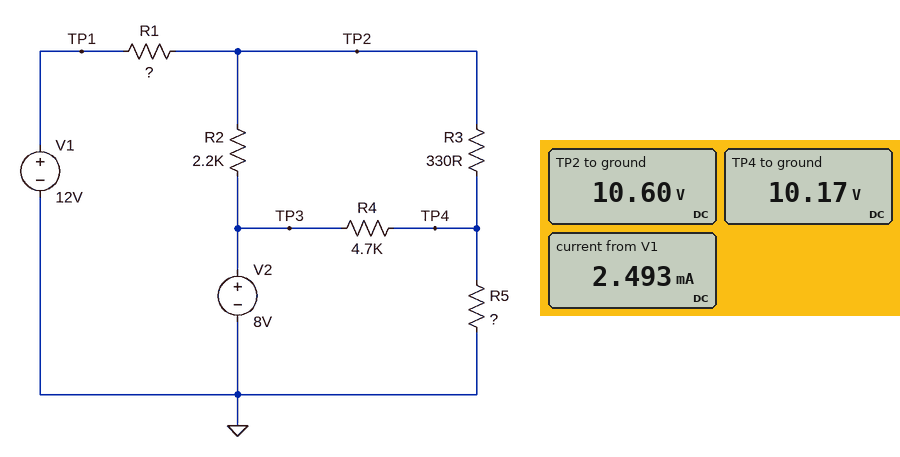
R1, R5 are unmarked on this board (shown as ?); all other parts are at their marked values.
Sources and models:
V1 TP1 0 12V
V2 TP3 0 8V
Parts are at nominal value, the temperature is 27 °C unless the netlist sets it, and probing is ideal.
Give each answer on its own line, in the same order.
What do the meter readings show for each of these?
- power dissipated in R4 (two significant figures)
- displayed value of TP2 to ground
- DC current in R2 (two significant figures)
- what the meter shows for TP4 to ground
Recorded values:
1.0 mW
10.60 V
1.2 mA
10.17 V
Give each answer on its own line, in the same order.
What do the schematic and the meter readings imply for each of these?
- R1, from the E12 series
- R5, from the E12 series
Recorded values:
560 Ω
12 kΩ
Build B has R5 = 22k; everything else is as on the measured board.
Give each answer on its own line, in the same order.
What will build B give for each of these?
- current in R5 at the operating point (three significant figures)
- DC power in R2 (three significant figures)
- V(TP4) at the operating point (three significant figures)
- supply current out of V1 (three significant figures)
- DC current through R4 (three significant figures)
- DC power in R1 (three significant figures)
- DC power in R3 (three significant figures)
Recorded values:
474 µA
3.43 mW
10.4 V
2.24 mA
515 µA
2.80 mW
323 µW
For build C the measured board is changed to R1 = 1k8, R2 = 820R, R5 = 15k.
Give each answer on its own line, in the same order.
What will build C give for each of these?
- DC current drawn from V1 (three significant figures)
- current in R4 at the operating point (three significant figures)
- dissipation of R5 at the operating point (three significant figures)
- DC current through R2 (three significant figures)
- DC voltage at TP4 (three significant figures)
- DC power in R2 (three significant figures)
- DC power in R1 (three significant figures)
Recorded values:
1.75 mA
132 µA
4.95 mW
1.04 mA
8.62 V
889 µW
5.50 mW
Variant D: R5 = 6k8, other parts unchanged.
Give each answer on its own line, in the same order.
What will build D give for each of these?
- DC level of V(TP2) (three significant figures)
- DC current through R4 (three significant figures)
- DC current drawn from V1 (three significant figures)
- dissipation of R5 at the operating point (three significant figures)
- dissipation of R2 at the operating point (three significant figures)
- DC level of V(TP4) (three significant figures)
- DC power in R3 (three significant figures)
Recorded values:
10.4 V
378 µA
2.90 mA
14.1 mW
2.57 mW
9.78 V
1.09 mW
